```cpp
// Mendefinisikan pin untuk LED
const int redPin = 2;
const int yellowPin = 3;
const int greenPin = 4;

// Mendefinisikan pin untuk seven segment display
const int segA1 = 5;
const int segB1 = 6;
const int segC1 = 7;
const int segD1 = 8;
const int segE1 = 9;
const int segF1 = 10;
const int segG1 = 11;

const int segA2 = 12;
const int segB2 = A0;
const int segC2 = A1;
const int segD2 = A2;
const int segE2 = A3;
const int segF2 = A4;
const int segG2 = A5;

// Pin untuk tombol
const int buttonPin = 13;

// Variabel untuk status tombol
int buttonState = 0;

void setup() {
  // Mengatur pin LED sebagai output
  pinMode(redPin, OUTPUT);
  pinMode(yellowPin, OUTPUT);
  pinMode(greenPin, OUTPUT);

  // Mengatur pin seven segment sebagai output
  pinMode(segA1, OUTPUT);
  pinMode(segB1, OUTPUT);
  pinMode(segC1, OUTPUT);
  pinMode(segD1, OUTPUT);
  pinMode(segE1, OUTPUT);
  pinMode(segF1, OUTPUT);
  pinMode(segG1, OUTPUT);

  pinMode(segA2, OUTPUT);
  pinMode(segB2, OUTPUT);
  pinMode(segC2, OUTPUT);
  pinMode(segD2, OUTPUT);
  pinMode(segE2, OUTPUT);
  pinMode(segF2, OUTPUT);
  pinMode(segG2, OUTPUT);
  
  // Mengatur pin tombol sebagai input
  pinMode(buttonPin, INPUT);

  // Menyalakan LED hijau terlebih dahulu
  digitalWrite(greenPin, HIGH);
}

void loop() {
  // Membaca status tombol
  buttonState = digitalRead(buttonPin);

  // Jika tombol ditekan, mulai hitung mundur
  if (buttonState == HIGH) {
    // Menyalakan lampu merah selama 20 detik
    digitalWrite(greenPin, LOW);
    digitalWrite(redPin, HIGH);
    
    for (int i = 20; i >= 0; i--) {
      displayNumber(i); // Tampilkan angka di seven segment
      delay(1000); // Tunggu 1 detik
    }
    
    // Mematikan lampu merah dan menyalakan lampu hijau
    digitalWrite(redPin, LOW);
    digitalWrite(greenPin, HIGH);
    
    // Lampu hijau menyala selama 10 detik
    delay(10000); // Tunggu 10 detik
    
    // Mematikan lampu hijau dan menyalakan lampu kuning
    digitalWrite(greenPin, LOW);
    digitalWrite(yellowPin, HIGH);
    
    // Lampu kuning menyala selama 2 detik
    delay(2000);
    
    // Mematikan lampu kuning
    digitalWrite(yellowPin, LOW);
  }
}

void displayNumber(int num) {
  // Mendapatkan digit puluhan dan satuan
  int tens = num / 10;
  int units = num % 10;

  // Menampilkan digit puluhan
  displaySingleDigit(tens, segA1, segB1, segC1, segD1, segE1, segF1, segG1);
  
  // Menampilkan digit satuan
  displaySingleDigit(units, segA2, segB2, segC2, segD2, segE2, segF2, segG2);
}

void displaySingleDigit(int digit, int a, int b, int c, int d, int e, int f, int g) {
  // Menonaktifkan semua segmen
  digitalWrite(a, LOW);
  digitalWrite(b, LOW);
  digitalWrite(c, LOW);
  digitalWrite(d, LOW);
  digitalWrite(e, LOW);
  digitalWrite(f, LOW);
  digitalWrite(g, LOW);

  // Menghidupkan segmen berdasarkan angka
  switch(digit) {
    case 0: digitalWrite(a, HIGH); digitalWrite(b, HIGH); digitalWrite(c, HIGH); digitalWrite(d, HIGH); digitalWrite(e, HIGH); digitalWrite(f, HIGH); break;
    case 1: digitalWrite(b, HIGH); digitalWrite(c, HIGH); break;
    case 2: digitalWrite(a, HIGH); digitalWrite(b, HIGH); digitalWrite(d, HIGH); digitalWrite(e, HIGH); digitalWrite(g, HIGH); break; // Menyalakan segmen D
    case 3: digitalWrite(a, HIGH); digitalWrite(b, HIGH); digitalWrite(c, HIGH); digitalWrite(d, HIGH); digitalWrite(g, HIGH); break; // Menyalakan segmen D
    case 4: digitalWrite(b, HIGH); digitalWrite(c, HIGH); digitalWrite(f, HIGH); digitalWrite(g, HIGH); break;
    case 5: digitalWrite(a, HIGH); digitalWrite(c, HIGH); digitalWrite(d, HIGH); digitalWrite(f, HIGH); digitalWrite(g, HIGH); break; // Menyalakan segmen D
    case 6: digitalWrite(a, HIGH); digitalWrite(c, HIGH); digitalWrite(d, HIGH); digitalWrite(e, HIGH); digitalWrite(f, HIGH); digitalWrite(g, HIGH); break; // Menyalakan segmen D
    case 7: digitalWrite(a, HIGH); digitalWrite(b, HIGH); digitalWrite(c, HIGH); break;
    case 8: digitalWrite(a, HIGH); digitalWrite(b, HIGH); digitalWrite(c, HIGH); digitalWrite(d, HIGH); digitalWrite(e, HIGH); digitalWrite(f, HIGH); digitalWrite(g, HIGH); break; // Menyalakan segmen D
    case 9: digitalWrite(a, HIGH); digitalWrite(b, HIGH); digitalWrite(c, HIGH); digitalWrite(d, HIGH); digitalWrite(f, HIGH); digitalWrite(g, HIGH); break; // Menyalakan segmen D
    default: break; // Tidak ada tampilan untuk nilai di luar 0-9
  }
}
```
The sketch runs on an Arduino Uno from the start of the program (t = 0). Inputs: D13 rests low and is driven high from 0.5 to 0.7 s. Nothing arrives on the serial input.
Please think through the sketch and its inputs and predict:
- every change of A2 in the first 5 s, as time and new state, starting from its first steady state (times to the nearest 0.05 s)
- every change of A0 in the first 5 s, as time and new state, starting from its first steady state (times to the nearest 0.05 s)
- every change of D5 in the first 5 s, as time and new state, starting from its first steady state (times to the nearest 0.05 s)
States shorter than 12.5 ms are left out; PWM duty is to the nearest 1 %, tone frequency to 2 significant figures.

0 s low; 0.5 s high; 3.5 s low; 4.5 s high
0 s low; 0.5 s high; 4.5 s low
0 s low; 0.5 s high; 1.5 s low
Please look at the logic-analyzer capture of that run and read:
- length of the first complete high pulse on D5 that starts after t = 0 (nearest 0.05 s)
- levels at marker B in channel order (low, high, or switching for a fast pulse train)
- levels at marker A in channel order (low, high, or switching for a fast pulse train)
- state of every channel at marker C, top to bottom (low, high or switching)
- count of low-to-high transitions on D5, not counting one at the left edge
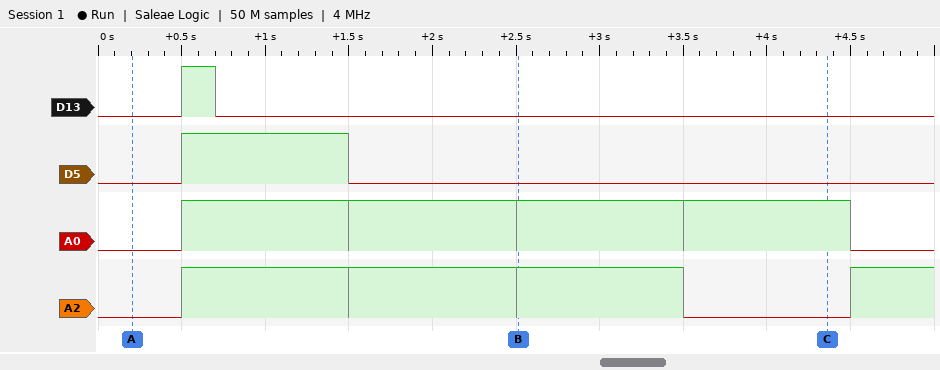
1.00 s
D13 low, D5 low, A0 high, A2 high
D13 low, D5 low, A0 low, A2 low
D13 low, D5 low, A0 high, A2 low
1
